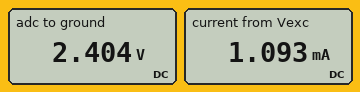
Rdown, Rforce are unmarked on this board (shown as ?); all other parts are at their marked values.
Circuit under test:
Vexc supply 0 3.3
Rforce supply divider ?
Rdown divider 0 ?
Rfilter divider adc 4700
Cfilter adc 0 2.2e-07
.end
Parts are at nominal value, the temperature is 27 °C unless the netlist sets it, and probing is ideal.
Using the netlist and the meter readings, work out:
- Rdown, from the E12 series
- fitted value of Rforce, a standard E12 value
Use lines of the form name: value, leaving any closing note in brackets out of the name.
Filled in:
Rdown, from the E12 series: 2.2 kΩ
fitted value of Rforce, a standard E12 value: 820 Ω
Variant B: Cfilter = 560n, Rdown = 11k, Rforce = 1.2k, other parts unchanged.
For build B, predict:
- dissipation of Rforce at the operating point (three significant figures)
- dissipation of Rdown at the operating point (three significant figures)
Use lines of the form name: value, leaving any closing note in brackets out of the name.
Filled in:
dissipation of Rforce at the operating point: 87.8 µW
dissipation of Rdown at the operating point: 805 µW
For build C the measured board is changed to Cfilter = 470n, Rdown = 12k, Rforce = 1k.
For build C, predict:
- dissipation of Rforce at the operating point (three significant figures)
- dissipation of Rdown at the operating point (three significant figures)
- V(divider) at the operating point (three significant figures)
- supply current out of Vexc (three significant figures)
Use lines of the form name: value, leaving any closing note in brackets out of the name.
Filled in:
dissipation of Rforce at the operating point: 64.4 µW
dissipation of Rdown at the operating point: 773 µW
V(divider) at the operating point: 3.05 V
supply current out of Vexc: 254 µA
